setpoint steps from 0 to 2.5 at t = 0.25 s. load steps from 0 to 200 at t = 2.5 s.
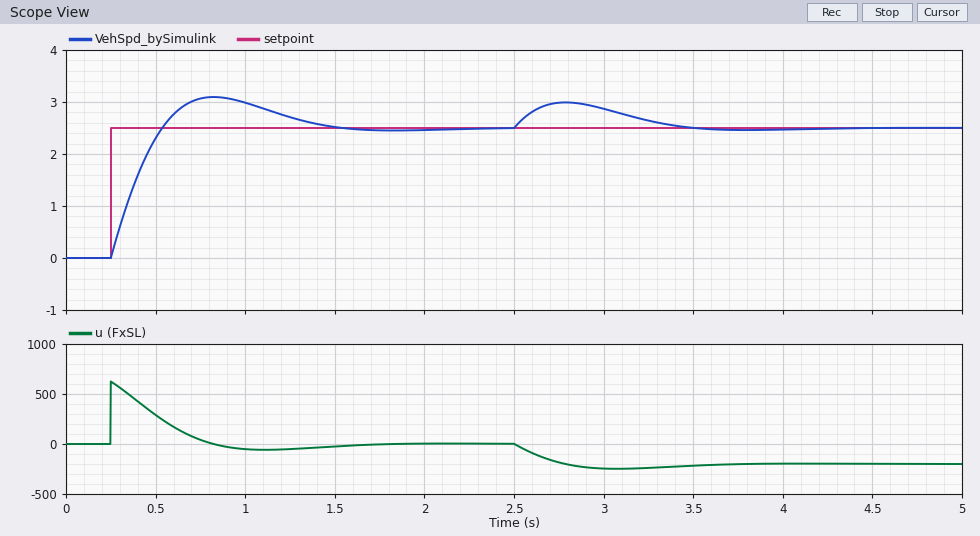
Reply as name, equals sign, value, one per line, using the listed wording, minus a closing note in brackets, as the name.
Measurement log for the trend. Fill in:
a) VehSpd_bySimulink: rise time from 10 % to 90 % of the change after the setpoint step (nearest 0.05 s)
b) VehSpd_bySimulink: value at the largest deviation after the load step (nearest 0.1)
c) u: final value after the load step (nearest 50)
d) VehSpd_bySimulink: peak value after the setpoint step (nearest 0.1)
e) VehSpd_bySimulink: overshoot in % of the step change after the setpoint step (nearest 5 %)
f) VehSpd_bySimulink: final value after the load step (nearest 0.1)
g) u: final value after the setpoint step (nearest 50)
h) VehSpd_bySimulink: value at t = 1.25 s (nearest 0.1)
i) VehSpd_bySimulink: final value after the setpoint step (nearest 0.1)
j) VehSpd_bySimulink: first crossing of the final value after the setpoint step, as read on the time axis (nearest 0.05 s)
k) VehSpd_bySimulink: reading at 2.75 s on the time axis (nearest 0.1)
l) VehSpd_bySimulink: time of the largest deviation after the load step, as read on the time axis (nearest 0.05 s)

VehSpd_bySimulink: rise time from 10 % to 90 % of the change after the setpoint step = 0.20 s
VehSpd_bySimulink: value at the largest deviation after the load step = 3.0
u: final value after the load step = -200
VehSpd_bySimulink: peak value after the setpoint step = 3.1
VehSpd_bySimulink: overshoot in % of the step change after the setpoint step = 25 %
VehSpd_bySimulink: final value after the load step = 2.5
u: final value after the setpoint step = 0
VehSpd_bySimulink: value at t = 1.25 s = 2.7
VehSpd_bySimulink: final value after the setpoint step = 2.5
VehSpd_bySimulink: first crossing of the final value after the setpoint step, as read on the time axis = 0.55 s
VehSpd_bySimulink: reading at 2.75 s on the time axis = 3.0
VehSpd_bySimulink: time of the largest deviation after the load step, as read on the time axis = 2.80 s
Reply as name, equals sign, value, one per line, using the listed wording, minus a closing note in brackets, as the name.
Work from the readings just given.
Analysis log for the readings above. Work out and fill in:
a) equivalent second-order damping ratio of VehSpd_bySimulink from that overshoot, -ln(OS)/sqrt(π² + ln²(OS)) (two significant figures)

equivalent second-order damping ratio of VehSpd_bySimulink from that overshoot, -ln(OS)/sqrt(π² + ln²(OS)) = 0.40
